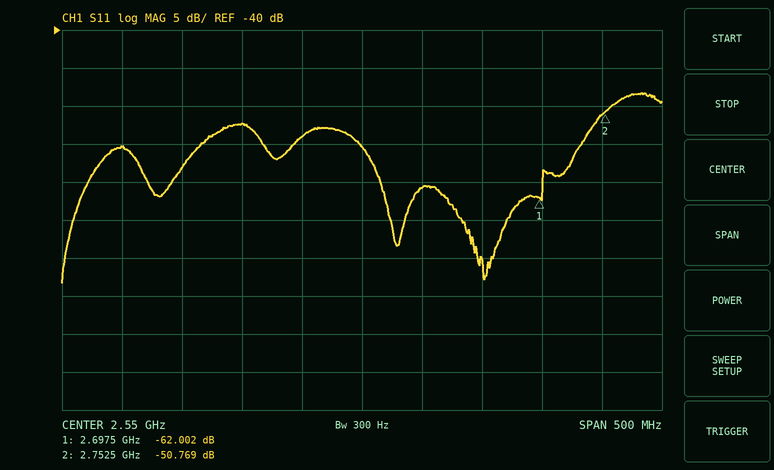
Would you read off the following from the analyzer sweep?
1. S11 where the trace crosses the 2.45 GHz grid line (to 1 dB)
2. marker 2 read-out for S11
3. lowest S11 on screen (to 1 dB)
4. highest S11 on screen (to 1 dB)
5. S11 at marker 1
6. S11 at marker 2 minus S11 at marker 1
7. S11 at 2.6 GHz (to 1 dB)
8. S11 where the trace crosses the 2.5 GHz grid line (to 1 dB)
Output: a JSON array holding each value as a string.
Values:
["-52 dB", "-50.769 dB", "-73 dB", "-48 dB", "-62.002 dB", "11.233 dB", "-61 dB", "-54 dB"]
